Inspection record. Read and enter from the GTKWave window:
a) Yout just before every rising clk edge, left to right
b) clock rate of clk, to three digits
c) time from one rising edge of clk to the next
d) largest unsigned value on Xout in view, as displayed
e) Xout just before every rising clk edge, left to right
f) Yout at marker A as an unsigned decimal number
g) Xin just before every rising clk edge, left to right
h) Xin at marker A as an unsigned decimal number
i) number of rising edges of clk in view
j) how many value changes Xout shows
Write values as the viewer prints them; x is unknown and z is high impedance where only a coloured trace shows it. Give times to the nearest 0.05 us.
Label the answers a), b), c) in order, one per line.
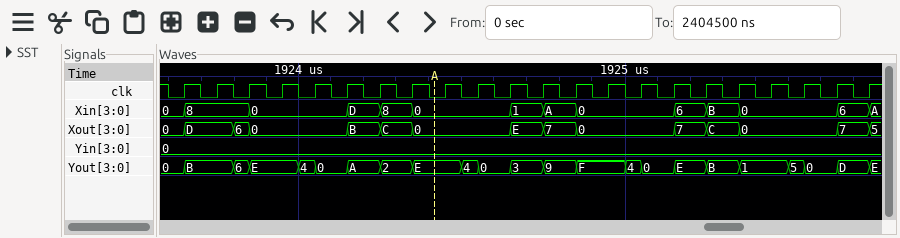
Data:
a) 0, B, 6, E, 4, 0, A, 2, E, 4, 0, 3, 9, F, 4, 0, E, B, 1, 5, 0, D
b) 10.0 MHz
c) 0.1 us
d) E
e) 0, D, 6, 0, 0, 0, B, C, 0, 0, 0, E, 7, 0, 0, 0, 7, C, 0, 0, 0, 7
f) 14
g) 0, 8, 8, 0, 0, 0, D, 8, 0, 0, 0, 1, A, 0, 0, 0, 6, B, 0, 0, 0, 6
h) 0
i) 22
j) 14
